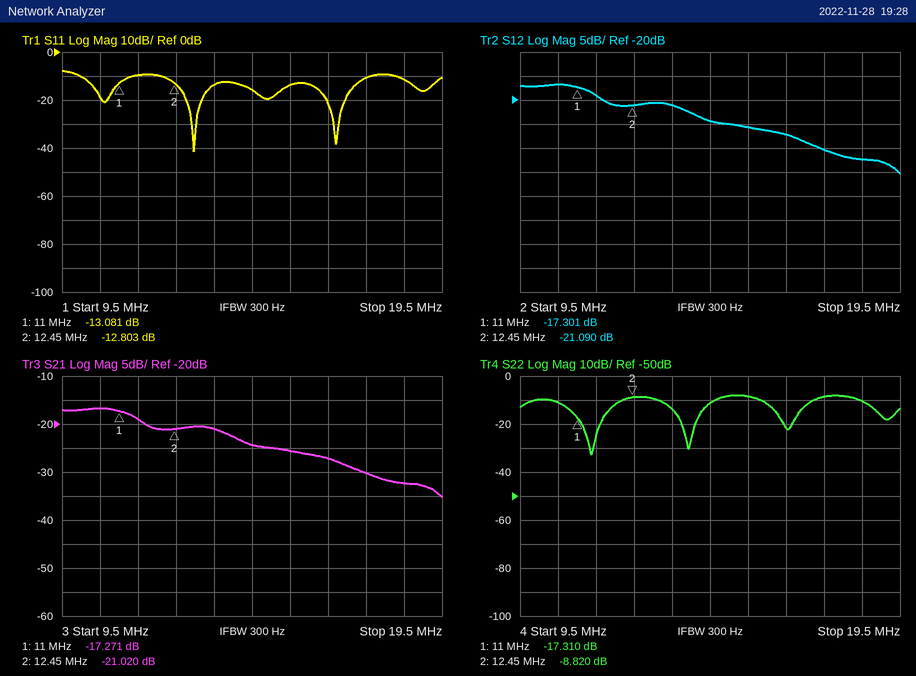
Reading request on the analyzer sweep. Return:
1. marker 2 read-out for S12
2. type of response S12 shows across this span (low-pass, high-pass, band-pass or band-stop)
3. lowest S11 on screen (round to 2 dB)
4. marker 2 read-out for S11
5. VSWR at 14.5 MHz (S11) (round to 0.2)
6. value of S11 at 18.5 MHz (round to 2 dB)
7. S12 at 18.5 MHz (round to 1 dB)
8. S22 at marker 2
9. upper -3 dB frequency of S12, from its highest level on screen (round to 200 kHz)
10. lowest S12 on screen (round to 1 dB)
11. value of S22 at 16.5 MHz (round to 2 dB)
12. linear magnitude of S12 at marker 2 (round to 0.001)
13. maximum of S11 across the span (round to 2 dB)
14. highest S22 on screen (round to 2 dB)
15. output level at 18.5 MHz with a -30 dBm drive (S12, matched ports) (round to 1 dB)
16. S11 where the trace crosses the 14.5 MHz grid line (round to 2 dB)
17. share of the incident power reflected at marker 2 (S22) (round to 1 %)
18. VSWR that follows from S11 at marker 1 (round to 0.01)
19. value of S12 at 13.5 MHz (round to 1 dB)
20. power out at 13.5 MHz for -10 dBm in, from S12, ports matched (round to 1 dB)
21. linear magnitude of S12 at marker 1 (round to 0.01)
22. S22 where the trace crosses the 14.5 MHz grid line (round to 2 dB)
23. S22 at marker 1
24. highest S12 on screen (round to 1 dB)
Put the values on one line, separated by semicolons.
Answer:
-21.090 dB; low-pass; -42 dB; -12.803 dB; 1.4; -12 dB; -32 dB; -8.820 dB; 11.6 MHz; -35 dB; -22 dB; 0.088; -8 dB; -8 dB; -62 dBm; -16 dB; 13 %; 1.57; -21 dB; -31 dBm; 0.14; -12 dB; -17.310 dB; -17 dB
